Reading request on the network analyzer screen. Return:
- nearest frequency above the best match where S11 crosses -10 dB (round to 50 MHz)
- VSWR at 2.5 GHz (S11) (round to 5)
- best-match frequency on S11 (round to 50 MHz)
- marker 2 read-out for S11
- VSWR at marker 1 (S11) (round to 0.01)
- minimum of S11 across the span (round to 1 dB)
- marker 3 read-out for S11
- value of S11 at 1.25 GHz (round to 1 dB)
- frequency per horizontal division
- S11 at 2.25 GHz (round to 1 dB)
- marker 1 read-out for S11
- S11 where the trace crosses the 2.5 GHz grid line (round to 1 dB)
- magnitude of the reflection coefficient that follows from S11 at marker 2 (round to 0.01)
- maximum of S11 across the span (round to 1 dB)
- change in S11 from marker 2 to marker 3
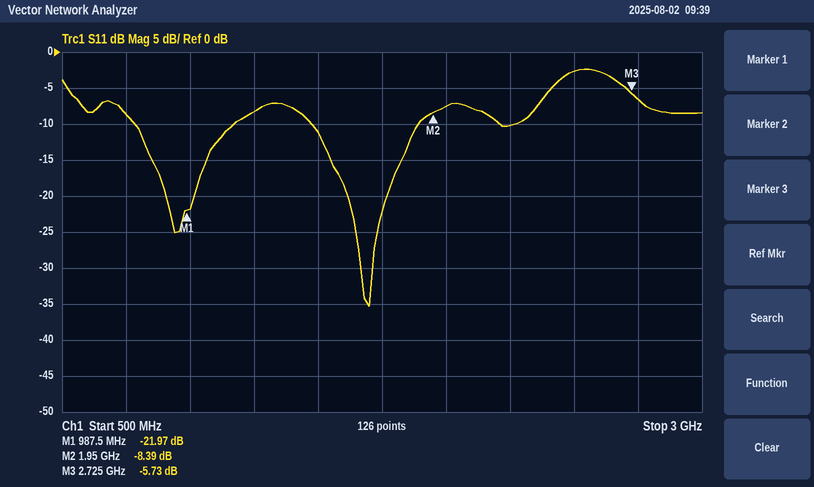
1.90 GHz
5
1.70 GHz
-8.39 dB
1.17
-35 dB
-5.73 dB
-8 dB
250 MHz
-10 dB
-21.97 dB
-3 dB
0.38
-2 dB
2.66 dB
